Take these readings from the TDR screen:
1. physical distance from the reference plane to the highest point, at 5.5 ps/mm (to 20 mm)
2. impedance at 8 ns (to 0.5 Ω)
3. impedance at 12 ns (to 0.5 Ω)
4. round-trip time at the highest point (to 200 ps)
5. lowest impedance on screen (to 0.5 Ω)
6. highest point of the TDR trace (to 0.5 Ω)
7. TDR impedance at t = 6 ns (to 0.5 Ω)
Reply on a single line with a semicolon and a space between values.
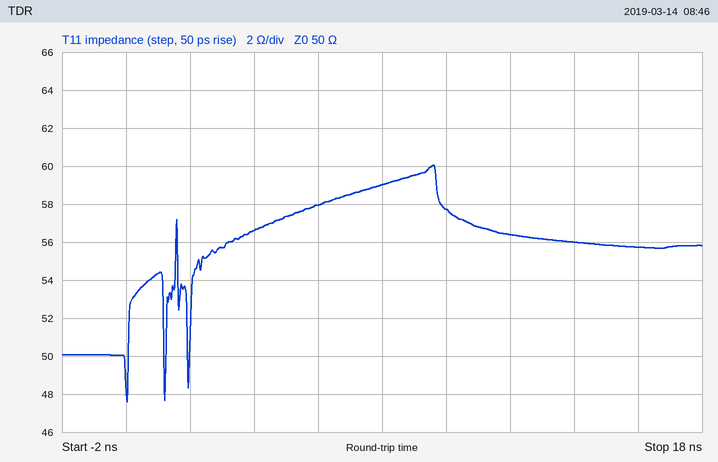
880 mm; 59.0 Ω; 56.5 Ω; 9.6 ns; 47.5 Ω; 60.0 Ω; 58.0 Ω
